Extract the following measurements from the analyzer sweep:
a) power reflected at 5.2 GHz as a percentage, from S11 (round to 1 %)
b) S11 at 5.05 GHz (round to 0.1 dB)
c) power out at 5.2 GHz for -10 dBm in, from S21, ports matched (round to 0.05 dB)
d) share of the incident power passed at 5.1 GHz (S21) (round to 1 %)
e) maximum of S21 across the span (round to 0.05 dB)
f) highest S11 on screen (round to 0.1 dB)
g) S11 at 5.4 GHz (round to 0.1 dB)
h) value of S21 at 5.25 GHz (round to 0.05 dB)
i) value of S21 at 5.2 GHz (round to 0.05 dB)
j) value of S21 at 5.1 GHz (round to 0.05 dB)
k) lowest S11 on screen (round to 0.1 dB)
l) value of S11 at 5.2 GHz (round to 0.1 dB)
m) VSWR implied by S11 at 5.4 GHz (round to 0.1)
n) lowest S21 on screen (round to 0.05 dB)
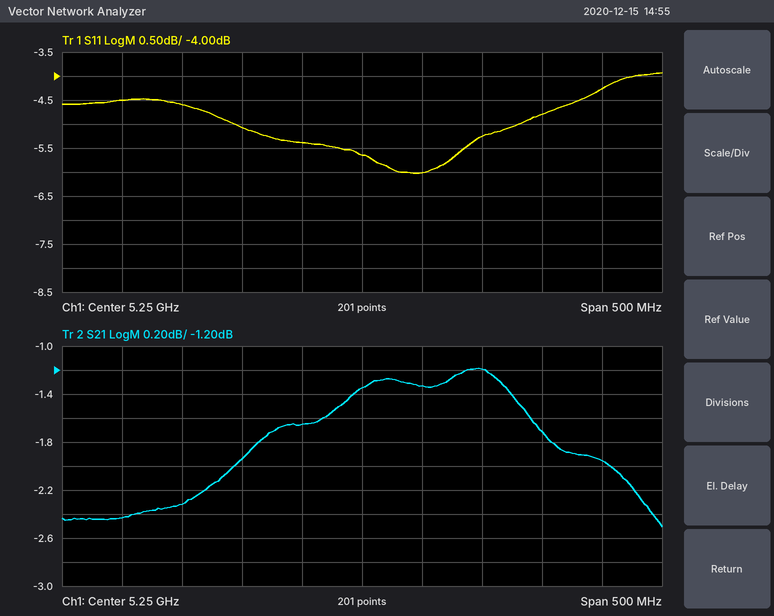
29 %
-4.5 dB
-11.65 dBm
59 %
-1.20 dB
-3.9 dB
-4.8 dB
-1.35 dB
-1.65 dB
-2.30 dB
-6.0 dB
-5.4 dB
3.7
-2.50 dB
